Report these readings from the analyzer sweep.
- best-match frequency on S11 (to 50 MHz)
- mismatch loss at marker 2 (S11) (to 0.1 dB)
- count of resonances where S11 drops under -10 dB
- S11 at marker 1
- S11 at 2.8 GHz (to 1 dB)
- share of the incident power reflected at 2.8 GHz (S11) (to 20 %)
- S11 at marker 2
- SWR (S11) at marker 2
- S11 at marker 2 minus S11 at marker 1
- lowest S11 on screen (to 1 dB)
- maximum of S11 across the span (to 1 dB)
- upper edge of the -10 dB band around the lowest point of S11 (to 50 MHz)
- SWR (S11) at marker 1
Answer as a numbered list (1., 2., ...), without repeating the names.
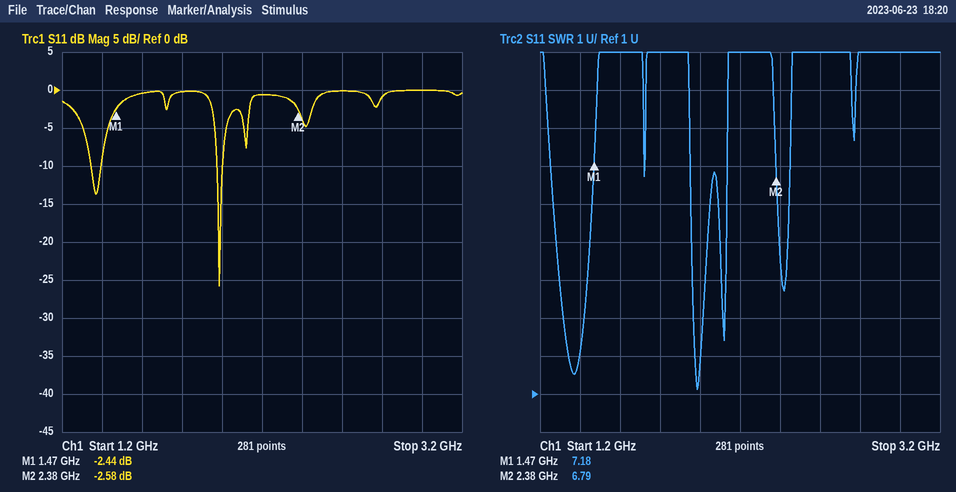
1. 2.00 GHz
2. 3.5 dB
3. 2
4. -2.44 dB
5. -1 dB
6. 80 %
7. -2.58 dB
8. 6.79
9. -0.14 dB
10. -26 dB
11. 0 dB
12. 2.00 GHz
13. 7.18
